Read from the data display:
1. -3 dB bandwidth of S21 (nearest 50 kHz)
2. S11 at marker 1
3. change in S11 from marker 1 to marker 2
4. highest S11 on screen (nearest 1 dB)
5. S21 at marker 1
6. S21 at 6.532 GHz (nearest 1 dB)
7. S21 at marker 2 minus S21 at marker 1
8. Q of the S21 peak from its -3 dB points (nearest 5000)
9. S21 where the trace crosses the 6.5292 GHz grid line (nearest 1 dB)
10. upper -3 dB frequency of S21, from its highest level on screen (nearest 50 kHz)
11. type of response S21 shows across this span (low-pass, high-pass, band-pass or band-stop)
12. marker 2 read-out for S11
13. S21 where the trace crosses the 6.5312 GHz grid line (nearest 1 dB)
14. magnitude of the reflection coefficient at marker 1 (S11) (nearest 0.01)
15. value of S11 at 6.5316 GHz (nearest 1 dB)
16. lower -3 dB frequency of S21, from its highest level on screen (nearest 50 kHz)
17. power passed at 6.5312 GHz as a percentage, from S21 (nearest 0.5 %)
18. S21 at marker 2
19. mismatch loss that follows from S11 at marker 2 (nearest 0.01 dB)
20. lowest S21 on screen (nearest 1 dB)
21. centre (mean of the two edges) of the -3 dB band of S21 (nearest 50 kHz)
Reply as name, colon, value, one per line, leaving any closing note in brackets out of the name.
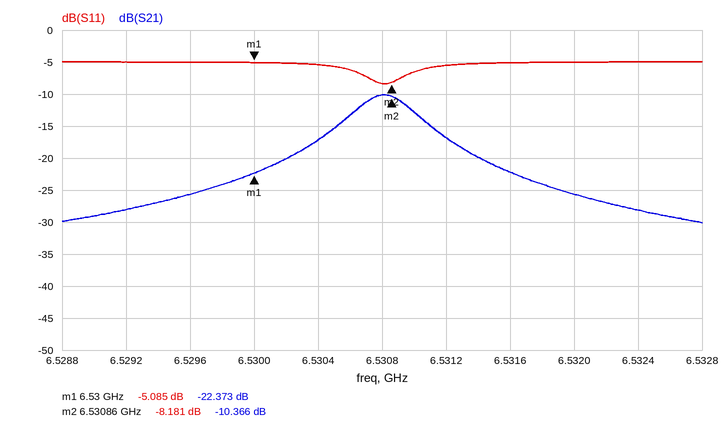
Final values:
-3 dB bandwidth of S21: 400 kHz
S11 at marker 1: -5.085 dB
change in S11 from marker 1 to marker 2: -3.096 dB
highest S11 on screen: -5 dB
S21 at marker 1: -22.373 dB
S21 at 6.532 GHz: -26 dB
S21 at marker 2 minus S21 at marker 1: 12.007 dB
Q of the S21 peak from its -3 dB points: 15000
S21 where the trace crosses the 6.5292 GHz grid line: -28 dB
upper -3 dB frequency of S21, from its highest level on screen: 6.53100 GHz
type of response S21 shows across this span: band-pass
marker 2 read-out for S11: -8.181 dB
S21 where the trace crosses the 6.5312 GHz grid line: -17 dB
magnitude of the reflection coefficient at marker 1 (S11): 0.56
value of S11 at 6.5316 GHz: -5 dB
lower -3 dB frequency of S21, from its highest level on screen: 6.53060 GHz
power passed at 6.5312 GHz as a percentage, from S21: 2.0 %
S21 at marker 2: -10.366 dB
mismatch loss that follows from S11 at marker 2: 0.72 dB
lowest S21 on screen: -30 dB
centre (mean of the two edges) of the -3 dB band of S21: 6.53080 GHz
